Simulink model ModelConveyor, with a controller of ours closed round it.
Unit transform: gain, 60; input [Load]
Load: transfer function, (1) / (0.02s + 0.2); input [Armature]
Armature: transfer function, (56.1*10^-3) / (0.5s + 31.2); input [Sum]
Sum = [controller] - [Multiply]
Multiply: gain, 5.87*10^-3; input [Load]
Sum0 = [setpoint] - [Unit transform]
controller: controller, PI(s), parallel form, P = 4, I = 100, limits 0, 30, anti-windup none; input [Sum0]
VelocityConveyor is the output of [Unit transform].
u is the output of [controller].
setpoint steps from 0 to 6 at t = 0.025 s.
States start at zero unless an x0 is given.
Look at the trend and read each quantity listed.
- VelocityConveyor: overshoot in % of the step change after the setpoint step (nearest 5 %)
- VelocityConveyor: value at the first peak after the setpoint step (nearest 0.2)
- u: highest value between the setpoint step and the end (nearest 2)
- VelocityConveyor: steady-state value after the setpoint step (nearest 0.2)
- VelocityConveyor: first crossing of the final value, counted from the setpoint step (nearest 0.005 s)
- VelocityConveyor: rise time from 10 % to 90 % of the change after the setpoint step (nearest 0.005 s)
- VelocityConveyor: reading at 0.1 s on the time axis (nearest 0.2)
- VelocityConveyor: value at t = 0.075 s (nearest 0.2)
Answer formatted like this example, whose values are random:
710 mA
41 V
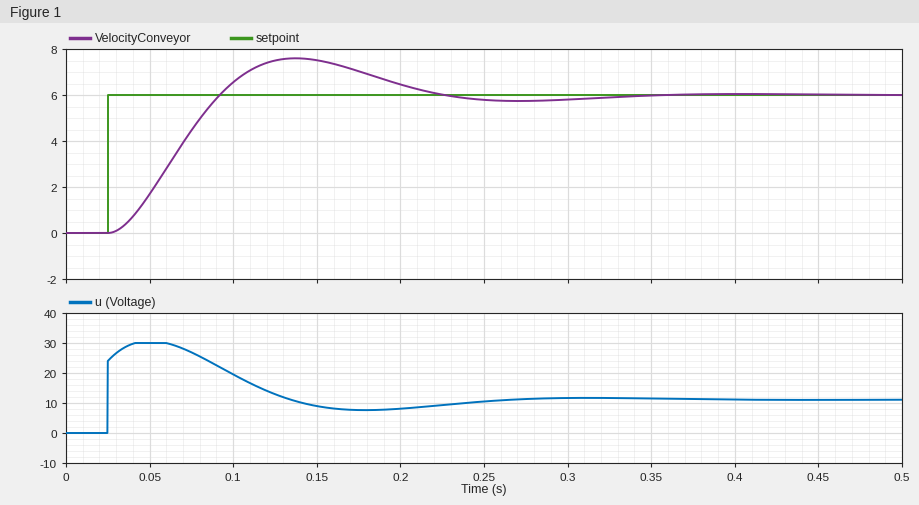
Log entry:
25 %
7.6
30
6.0
0.065 s
0.045 s
6.6
4.4
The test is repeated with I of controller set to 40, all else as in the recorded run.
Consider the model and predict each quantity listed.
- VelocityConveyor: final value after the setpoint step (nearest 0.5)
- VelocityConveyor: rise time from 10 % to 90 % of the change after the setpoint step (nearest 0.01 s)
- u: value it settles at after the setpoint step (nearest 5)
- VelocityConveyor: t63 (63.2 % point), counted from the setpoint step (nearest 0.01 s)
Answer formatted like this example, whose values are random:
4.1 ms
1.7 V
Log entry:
6.0
0.07 s
10
0.05 s
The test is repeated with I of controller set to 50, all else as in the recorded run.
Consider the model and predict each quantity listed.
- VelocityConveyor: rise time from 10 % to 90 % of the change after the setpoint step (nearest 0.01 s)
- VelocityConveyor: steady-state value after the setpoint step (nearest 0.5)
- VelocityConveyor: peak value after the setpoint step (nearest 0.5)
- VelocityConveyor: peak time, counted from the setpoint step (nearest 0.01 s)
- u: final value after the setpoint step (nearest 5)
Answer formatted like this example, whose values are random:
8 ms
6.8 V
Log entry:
0.06 s
6.0
6.5
0.14 s
10
